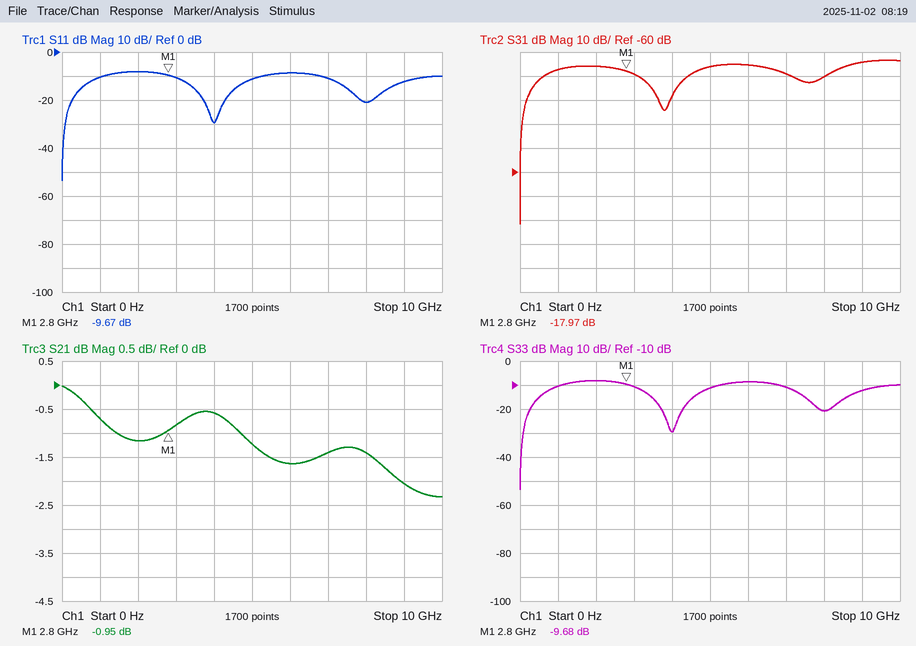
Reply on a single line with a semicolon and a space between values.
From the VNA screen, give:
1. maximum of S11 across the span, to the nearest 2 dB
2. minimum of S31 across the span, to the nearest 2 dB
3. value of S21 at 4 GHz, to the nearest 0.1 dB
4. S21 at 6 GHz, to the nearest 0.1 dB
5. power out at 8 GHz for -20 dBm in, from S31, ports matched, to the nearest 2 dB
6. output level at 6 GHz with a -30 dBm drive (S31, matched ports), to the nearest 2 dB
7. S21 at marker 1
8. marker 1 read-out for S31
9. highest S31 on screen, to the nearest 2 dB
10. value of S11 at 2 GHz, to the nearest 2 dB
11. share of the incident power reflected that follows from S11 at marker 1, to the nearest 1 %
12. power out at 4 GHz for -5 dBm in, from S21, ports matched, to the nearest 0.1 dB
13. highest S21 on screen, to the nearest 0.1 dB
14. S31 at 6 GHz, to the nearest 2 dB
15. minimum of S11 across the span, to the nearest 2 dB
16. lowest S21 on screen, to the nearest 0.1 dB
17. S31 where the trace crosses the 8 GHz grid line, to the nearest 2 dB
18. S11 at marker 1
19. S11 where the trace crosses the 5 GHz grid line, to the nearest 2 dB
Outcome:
-8 dB; -82 dB; -0.6 dB; -1.6 dB; -40 dBm; -46 dBm; -0.95 dB; -17.97 dB; -14 dB; -8 dB; 11 %; -5.6 dBm; 0.0 dB; -16 dB; -54 dB; -2.3 dB; -20 dB; -9.67 dB; -12 dB
